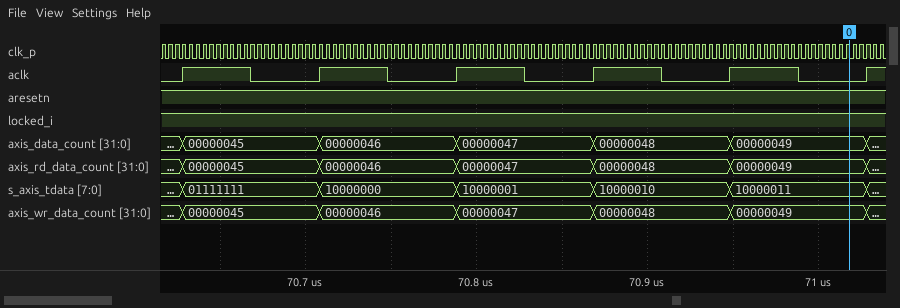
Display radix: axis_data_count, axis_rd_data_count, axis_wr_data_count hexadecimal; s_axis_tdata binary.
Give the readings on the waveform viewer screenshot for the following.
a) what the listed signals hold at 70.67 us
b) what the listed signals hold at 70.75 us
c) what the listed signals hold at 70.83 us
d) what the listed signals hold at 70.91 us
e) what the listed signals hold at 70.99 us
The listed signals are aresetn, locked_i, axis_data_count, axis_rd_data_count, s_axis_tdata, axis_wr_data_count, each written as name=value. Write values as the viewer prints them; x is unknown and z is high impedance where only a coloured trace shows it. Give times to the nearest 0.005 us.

aresetn=1, locked_i=1, axis_data_count=00000045, axis_rd_data_count=00000045, s_axis_tdata=01111111, axis_wr_data_count=00000045
aresetn=1, locked_i=1, axis_data_count=00000046, axis_rd_data_count=00000046, s_axis_tdata=10000000, axis_wr_data_count=00000046
aresetn=1, locked_i=1, axis_data_count=00000047, axis_rd_data_count=00000047, s_axis_tdata=10000001, axis_wr_data_count=00000047
aresetn=1, locked_i=1, axis_data_count=00000048, axis_rd_data_count=00000048, s_axis_tdata=10000010, axis_wr_data_count=00000048
aresetn=1, locked_i=1, axis_data_count=00000049, axis_rd_data_count=00000049, s_axis_tdata=10000011, axis_wr_data_count=00000049
